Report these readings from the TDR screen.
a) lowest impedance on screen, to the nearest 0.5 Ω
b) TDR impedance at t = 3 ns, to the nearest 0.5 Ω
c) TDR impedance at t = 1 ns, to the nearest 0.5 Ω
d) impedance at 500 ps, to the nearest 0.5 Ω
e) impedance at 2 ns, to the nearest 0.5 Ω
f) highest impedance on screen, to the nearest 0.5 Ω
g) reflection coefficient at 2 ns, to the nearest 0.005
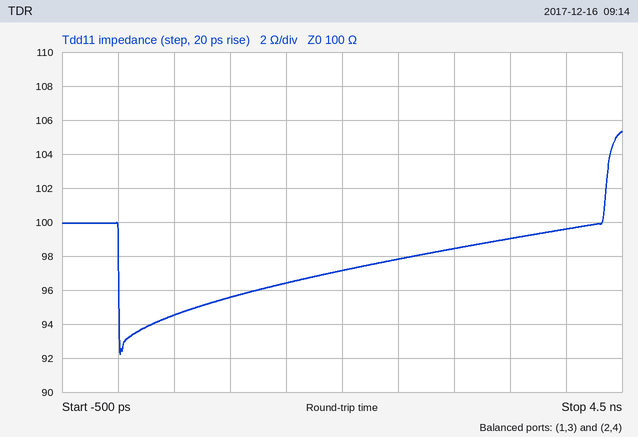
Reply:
92.0 Ω
98.5 Ω
95.5 Ω
94.5 Ω
97.0 Ω
105.5 Ω
-0.015
